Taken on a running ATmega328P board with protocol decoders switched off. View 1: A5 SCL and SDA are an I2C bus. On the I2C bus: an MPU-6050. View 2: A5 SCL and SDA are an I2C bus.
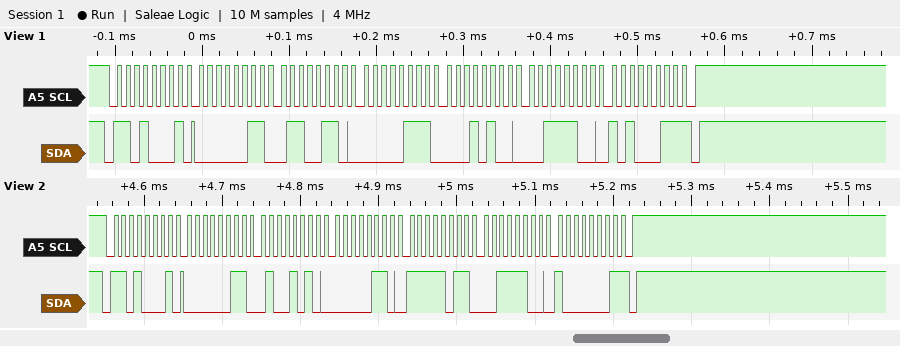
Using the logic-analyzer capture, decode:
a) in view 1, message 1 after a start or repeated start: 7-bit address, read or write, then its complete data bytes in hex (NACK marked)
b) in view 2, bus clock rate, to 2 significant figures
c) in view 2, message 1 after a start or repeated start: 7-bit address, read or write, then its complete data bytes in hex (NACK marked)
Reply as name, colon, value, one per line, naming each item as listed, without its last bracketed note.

in view 1, message 1 after a start or repeated start: 7-bit address, read or write, then its complete data bytes in hex: 0x68 read: 03 66 07 14 3C A3 NACK
in view 2, bus clock rate, to 2 significant figures: 100 kHz
in view 2, message 1 after a start or repeated start: 7-bit address, read or write, then its complete data bytes in hex: 0x68 read: 03 4A 06 FB 3C 81 NACK
